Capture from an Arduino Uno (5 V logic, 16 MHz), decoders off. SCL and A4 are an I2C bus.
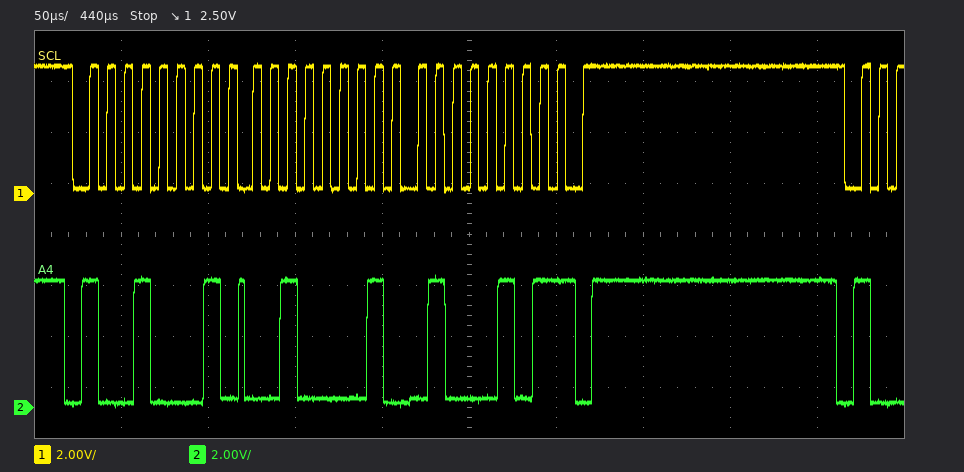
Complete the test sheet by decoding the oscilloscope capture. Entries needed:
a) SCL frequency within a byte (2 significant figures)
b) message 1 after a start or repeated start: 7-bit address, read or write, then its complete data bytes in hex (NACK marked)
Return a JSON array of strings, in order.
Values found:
["100 kHz", "0x48 read: 21 45 NACK"]
